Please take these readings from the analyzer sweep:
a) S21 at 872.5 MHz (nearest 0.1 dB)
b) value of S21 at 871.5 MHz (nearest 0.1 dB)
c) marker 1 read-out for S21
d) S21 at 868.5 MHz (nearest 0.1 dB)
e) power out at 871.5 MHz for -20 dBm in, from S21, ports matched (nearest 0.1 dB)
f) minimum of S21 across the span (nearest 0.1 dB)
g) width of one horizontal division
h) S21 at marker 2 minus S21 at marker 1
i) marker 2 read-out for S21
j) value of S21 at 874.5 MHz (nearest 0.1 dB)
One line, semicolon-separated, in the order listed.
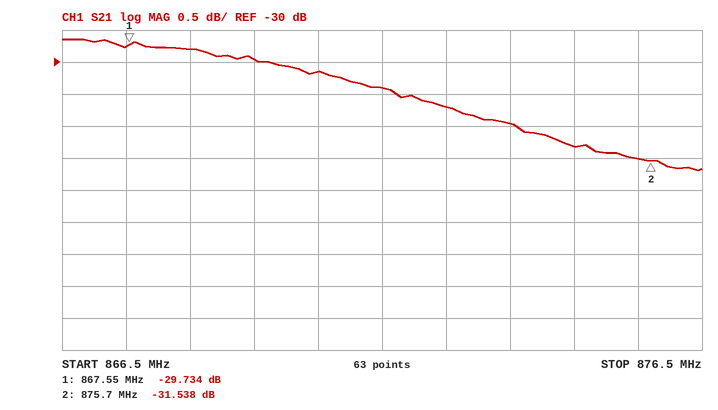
-30.7 dB; -30.4 dB; -29.734 dB; -29.8 dB; -50.4 dBm; -31.7 dB; 1 MHz; -1.804 dB; -31.538 dB; -31.3 dB
